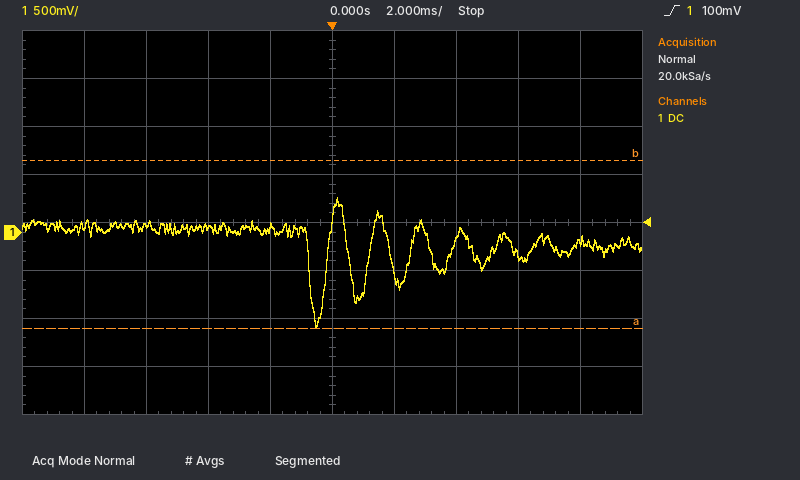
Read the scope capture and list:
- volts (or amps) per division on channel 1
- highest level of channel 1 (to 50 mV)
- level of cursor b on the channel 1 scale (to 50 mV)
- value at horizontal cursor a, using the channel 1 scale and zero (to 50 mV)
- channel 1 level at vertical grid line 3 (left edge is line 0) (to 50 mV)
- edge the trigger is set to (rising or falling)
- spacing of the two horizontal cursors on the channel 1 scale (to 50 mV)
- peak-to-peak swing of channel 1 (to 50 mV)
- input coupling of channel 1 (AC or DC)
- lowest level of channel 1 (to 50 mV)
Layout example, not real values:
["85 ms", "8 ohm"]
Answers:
["500 mV", "350 mV", "750 mV", "-1.00 V", "50 mV", "rising", "1.75 V", "1.35 V", "DC", "-1.00 V"]
